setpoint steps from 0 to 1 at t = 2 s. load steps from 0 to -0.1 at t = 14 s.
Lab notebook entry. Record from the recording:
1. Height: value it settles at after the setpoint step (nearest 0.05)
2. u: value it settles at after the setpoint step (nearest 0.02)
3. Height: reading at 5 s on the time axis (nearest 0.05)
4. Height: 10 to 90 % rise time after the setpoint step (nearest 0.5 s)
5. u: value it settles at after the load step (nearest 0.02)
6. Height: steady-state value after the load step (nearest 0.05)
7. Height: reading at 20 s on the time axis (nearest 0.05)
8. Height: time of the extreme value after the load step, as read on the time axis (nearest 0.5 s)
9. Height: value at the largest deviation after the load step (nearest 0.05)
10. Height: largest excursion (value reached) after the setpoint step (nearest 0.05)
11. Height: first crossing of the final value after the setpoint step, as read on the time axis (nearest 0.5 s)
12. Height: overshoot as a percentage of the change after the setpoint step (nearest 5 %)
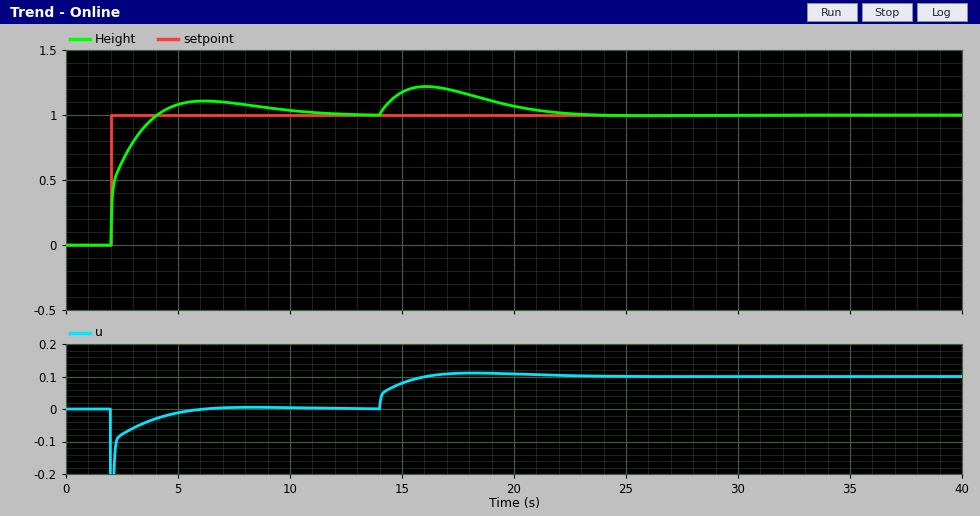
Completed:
1.00
0.00
1.10
1.5 s
0.10
1.00
1.05
16.0 s
1.20
1.10
4.0 s
10 %
